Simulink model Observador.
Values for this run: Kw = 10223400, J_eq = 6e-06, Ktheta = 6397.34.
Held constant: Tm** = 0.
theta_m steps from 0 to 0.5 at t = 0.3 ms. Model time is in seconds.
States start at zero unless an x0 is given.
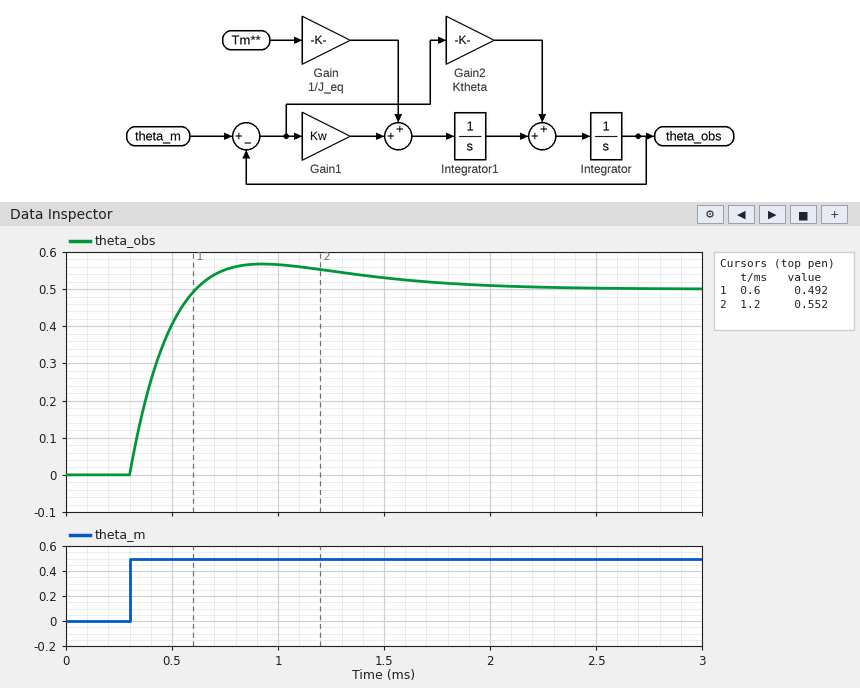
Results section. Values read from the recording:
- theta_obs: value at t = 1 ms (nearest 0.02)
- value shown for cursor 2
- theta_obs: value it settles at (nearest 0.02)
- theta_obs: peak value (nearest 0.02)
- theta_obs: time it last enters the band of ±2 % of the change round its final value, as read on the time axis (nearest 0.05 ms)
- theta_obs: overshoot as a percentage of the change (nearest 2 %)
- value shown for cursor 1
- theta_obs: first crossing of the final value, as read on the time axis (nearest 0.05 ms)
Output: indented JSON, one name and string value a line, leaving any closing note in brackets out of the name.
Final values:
{
  "theta_obs: value at t = 1 ms": "0.56",
  "value shown for cursor 2": "0.552",
  "theta_obs: value it settles at": "0.50",
  "theta_obs: peak value": "0.56",
  "theta_obs: time it last enters the band of ±2 % of the change round its final value, as read on the time axis": "2.00 ms",
  "theta_obs: overshoot as a percentage of the change": "14 %",
  "value shown for cursor 1": "0.492",
  "theta_obs: first crossing of the final value, as read on the time axis": "0.60 ms"
}
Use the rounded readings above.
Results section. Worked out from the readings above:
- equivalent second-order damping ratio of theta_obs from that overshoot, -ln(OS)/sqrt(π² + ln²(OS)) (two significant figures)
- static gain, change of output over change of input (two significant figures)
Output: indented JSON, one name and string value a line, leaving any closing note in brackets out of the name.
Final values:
{
  "equivalent second-order damping ratio of theta_obs from that overshoot, -ln(OS)/sqrt(π² + ln²(OS))": "0.53",
  "static gain, change of output over change of input": "1.0"
}
